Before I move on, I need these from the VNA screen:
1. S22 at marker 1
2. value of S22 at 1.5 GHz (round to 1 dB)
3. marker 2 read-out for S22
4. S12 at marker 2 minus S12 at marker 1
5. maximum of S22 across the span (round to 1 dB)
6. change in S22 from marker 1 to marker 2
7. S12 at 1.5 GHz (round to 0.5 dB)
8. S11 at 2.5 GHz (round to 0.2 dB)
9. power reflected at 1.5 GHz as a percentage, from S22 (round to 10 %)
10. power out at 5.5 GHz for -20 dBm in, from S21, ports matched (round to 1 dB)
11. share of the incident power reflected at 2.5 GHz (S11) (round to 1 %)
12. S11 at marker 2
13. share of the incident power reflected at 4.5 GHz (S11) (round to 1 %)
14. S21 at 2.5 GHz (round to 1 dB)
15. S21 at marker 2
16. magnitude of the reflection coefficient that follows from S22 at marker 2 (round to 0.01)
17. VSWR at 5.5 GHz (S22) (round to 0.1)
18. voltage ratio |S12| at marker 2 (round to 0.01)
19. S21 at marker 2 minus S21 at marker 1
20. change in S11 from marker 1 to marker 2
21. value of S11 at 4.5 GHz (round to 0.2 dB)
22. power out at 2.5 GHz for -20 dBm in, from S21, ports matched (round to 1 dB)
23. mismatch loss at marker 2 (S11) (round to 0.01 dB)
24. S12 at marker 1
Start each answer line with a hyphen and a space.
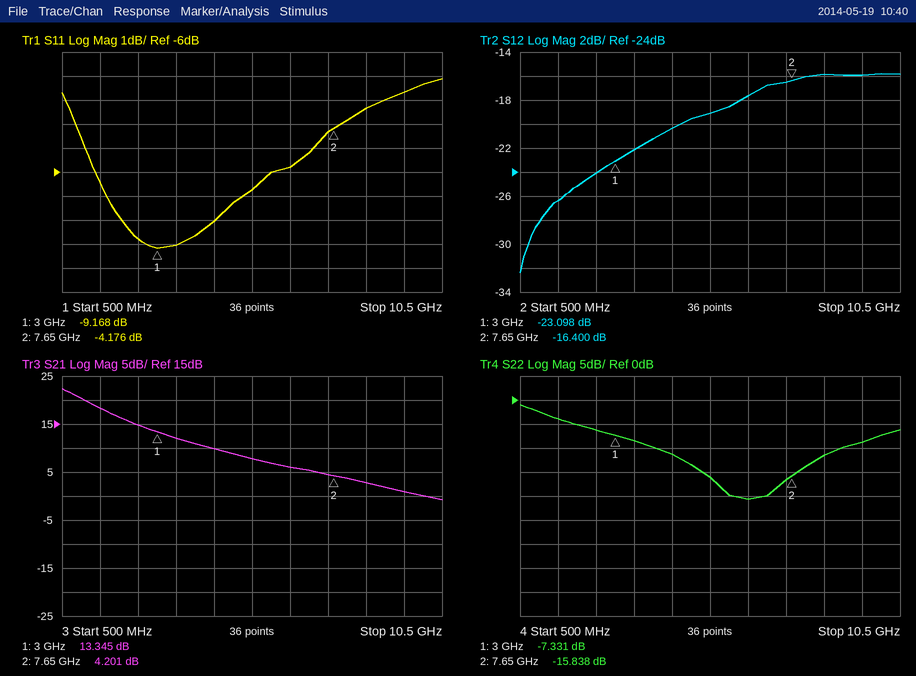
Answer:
- -7.331 dB
- -4 dB
- -15.838 dB
- 6.698 dB
- -1 dB
- -8.507 dB
- -26.5 dB
- -8.8 dB
- 40 %
- -12 dBm
- 13 %
- -4.176 dB
- 16 %
- 15 dB
- 4.201 dB
- 0.16
- 1.4
- 0.15
- -9.144 dB
- 4.992 dB
- -8.0 dB
- -5 dBm
- 2.09 dB
- -23.098 dB
